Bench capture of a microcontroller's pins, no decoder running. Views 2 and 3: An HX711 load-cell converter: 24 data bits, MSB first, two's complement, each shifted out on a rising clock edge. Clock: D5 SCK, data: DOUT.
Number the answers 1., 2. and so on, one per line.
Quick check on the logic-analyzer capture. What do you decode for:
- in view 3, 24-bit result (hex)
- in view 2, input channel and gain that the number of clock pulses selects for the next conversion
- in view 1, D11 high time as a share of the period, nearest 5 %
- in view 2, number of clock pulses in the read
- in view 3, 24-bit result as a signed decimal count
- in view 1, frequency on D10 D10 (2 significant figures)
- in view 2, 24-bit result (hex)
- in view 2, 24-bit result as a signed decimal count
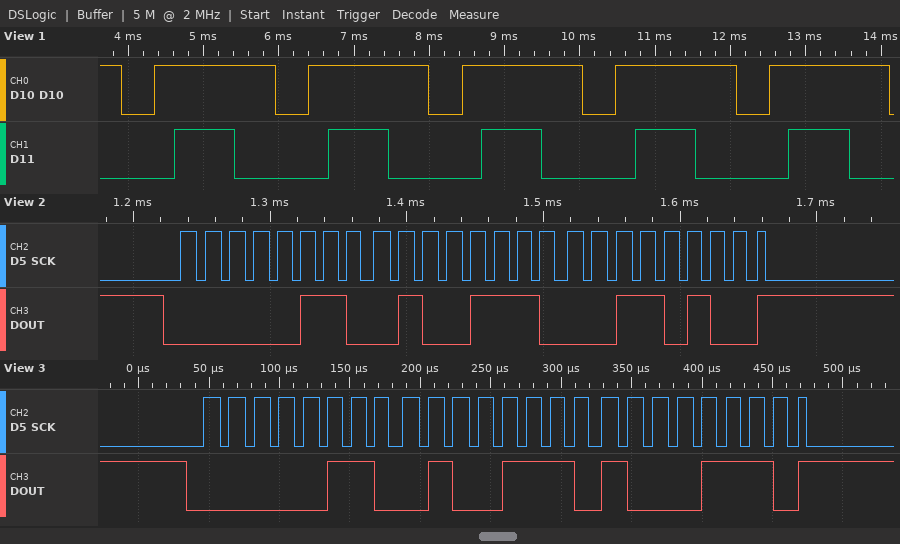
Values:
1. 0x064E8E
2. channel A, gain 128
3. 40 %
4. 25
5. 413326
6. 490 Hz
7. 0x064E34
8. 413236
